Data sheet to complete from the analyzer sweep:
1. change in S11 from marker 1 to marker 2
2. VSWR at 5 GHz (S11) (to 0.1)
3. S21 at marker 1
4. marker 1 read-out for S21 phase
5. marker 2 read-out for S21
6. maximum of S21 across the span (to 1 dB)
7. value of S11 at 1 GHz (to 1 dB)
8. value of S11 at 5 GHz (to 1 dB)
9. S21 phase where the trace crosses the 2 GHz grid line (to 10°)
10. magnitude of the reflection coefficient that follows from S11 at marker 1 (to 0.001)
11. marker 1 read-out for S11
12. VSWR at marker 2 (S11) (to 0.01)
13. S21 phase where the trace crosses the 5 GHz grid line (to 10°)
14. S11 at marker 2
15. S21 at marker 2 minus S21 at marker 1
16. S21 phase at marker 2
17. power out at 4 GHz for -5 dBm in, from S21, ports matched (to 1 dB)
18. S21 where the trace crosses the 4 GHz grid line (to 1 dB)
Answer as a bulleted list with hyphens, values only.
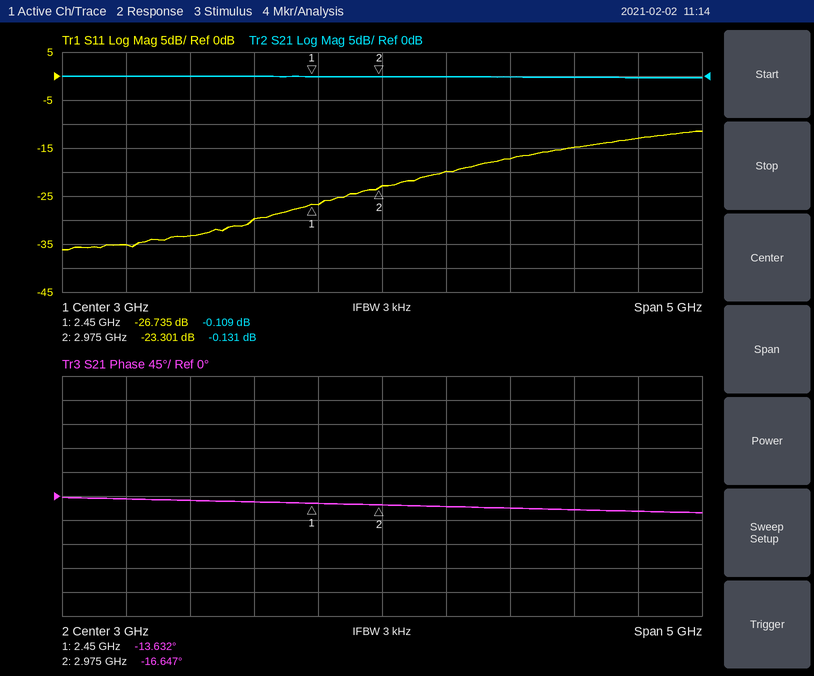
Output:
- 3.434 dB
- 1.6
- -0.109 dB
- -13.632°
- -0.131 dB
- 0 dB
- -35 dB
- -13 dB
- -10°
- 0.046
- -26.735 dB
- 1.15
- -30°
- -23.301 dB
- -0.022 dB
- -16.647°
- -5 dBm
- 0 dB
